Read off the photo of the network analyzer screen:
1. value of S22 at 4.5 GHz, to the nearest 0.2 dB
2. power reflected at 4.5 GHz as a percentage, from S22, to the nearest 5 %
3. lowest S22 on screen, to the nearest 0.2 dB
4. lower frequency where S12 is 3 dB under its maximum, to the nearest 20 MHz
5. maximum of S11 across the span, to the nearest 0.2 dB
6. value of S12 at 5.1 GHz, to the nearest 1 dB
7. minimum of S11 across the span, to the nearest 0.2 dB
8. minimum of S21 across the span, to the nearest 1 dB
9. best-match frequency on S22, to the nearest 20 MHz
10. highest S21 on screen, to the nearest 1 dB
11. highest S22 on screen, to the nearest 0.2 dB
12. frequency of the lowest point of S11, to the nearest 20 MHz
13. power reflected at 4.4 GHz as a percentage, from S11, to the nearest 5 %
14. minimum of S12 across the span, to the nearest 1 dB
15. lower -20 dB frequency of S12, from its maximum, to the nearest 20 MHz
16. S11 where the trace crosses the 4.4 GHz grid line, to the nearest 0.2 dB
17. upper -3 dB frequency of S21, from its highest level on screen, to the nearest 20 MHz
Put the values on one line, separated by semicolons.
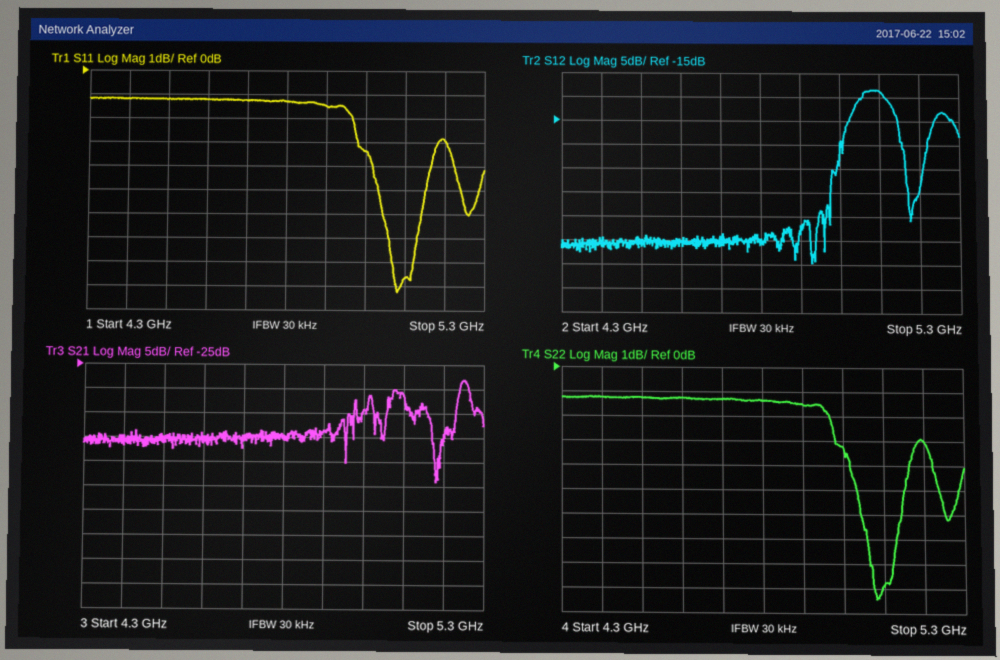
-1.2 dB; 75 %; -9.4 dB; 5.04 GHz; -1.2 dB; -9 dB; -9.2 dB; -49 dB; 5.08 GHz; -28 dB; -1.2 dB; 5.08 GHz; 75 %; -45 dB; 4.98 GHz; -1.2 dB; 5.26 GHz
